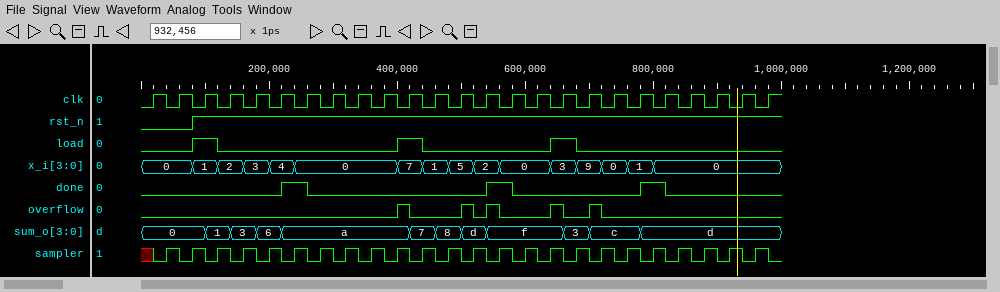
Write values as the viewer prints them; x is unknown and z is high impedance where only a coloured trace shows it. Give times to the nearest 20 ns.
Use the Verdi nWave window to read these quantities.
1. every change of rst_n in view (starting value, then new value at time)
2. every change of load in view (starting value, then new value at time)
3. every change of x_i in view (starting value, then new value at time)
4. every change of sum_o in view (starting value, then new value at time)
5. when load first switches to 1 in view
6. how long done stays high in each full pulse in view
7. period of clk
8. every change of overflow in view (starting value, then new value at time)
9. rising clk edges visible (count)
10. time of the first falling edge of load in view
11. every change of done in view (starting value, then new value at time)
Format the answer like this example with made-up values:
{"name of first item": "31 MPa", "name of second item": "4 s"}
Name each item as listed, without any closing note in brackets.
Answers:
{"every change of rst_n in view": "0, 1 at 80 ns", "every change of load in view": "0, 1 at 80 ns, 0 at 120 ns, 1 at 400 ns, 0 at 440 ns, 1 at 640 ns, 0 at 680 ns", "every change of x_i in view": "0, 1 at 80 ns, 2 at 120 ns, 3 at 160 ns, 4 at 200 ns, 0 at 240 ns, 7 at 400 ns, 1 at 440 ns, 5 at 480 ns, 2 at 520 ns, 0 at 560 ns, 3 at 640 ns, 9 at 680 ns, 0 at 720 ns, 1 at 760 ns, 0 at 800 ns", "every change of sum_o in view": "0, 1 at 100 ns, 3 at 140 ns, 6 at 180 ns, a at 220 ns, 7 at 420 ns, 8 at 460 ns, d at 500 ns, f at 540 ns, 3 at 660 ns, c at 700 ns, d at 780 ns", "when load first switches to 1 in view": "80 ns", "how long done stays high in each full pulse in view": "40 ns, 40 ns, 40 ns", "period of clk": "40 ns", "every change of overflow in view": "0, 1 at 400 ns, 0 at 420 ns, 1 at 500 ns, 0 at 520 ns, 1 at 540 ns, 0 at 560 ns, 1 at 640 ns, 0 at 660 ns, 1 at 700 ns, 0 at 720 ns", "rising clk edges visible": "25", "time of the first falling edge of load in view": "120 ns", "every change of done in view": "0, 1 at 220 ns, 0 at 260 ns, 1 at 540 ns, 0 at 580 ns, 1 at 780 ns, 0 at 820 ns"}
